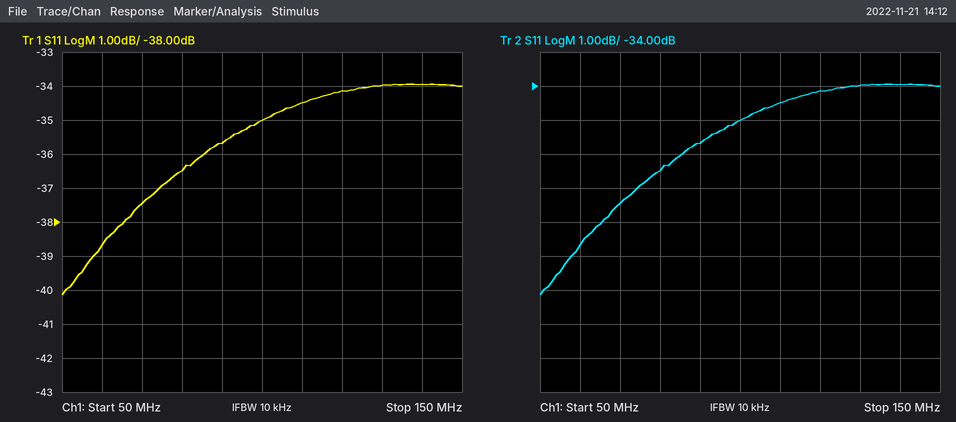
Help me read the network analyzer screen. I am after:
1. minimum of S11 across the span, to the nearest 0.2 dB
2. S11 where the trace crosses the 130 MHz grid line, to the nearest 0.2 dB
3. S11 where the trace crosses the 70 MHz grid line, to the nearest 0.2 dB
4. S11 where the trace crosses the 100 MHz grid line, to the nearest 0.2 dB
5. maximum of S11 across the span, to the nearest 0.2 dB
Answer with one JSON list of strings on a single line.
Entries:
["-40.2 dB", "-34.0 dB", "-37.4 dB", "-35.0 dB", "-34.0 dB"]
